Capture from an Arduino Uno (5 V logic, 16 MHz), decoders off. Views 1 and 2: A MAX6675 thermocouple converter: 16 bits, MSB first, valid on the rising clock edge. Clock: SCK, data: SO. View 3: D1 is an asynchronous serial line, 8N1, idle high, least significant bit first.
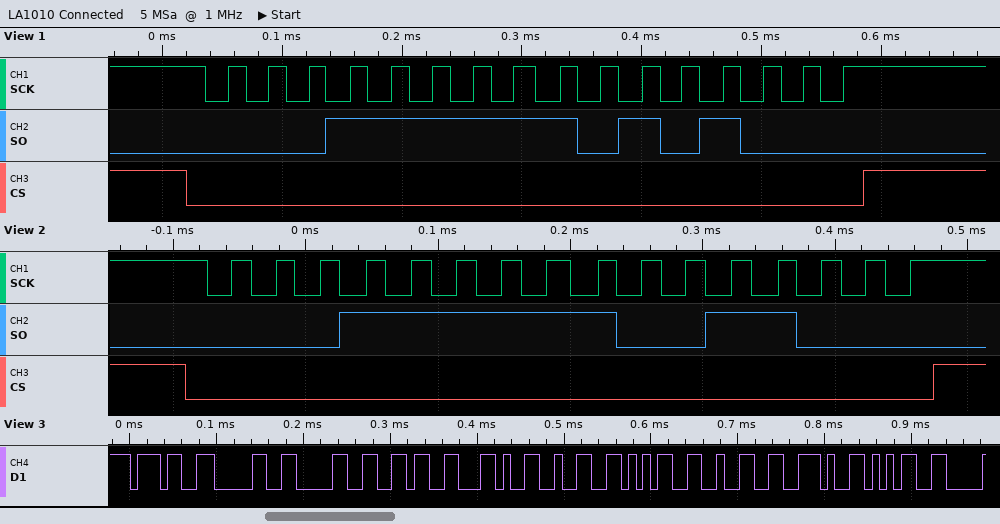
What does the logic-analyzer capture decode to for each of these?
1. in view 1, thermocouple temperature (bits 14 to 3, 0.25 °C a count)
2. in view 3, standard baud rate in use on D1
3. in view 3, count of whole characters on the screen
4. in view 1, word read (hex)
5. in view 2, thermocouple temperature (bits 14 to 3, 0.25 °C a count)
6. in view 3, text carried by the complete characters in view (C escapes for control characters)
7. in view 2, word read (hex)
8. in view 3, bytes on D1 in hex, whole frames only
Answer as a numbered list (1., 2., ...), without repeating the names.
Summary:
1. 253.25 °C
2. 115200 baud
3. 10
4. 0x1FA8
5. 252.75 °C
6. "7006,252.5"
7. 0x1F98
8. 37 30 30 36 2C 32 35 32 2E 35
